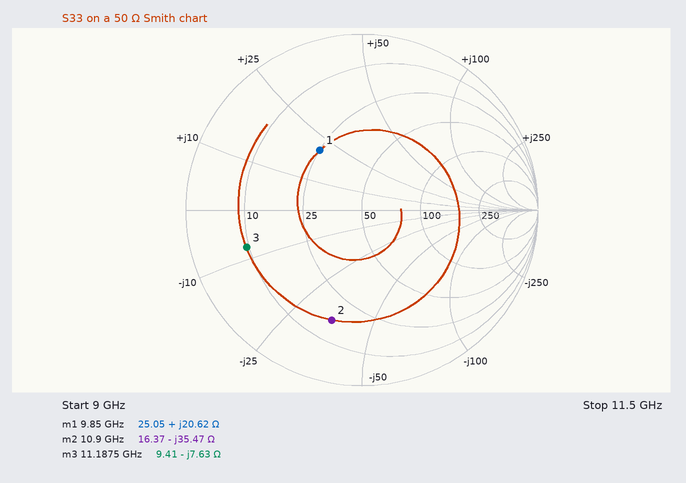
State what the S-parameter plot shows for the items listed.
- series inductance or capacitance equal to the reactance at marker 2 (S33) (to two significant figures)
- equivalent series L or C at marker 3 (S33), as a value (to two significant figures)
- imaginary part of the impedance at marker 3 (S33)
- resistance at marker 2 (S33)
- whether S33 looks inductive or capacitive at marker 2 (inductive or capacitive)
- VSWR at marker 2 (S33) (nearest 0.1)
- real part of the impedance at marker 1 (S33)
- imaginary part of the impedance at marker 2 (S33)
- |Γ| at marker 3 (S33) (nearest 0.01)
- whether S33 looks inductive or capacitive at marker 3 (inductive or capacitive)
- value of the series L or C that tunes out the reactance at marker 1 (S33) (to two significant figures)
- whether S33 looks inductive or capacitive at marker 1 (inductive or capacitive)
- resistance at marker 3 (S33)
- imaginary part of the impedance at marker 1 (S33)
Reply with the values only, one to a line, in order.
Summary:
410 fF
1.9 pF
-7.63 Ω
16.37 Ω
capacitive
4.7
25.05 Ω
-35.47 Ω
0.69
capacitive
780 fF
inductive
9.41 Ω
+20.62 Ω
